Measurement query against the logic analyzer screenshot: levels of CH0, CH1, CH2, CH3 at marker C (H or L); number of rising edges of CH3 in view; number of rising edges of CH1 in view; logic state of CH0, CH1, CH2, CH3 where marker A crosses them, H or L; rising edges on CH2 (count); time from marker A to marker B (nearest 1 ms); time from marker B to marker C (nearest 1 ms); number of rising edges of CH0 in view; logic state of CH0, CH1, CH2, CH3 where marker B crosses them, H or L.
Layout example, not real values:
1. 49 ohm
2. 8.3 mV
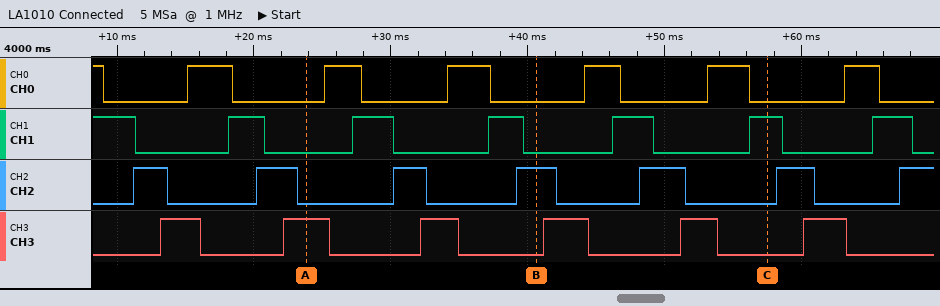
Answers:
1. CH0=L, CH1=H, CH2=L, CH3=L
2. 6
3. 6
4. CH0=L, CH1=L, CH2=L, CH3=H
5. 7
6. 17 ms
7. 17 ms
8. 6
9. CH0=L, CH1=L, CH2=H, CH3=L
